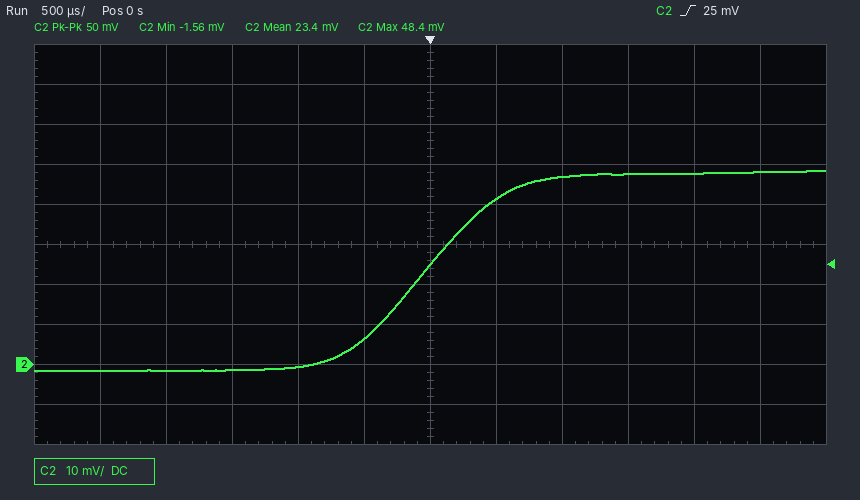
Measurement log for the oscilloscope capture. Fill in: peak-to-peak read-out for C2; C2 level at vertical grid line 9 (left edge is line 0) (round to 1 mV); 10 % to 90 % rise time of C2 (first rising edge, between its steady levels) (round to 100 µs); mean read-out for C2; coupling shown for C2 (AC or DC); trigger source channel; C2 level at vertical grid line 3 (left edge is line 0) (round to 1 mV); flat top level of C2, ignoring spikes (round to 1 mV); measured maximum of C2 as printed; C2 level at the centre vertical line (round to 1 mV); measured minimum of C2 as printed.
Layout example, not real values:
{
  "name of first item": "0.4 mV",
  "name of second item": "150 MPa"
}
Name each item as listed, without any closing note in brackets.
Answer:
{
  "peak-to-peak read-out for C2": "50 mV",
  "C2 level at vertical grid line 9 (left edge is line 0)": "48 mV",
  "10 % to 90 % rise time of C2 (first rising edge, between its steady levels)": "1.2 ms",
  "mean read-out for C2": "23.4 mV",
  "coupling shown for C2": "DC",
  "trigger source channel": "C2",
  "C2 level at vertical grid line 3 (left edge is line 0)": "-1 mV",
  "flat top level of C2, ignoring spikes": "48 mV",
  "measured maximum of C2 as printed": "48.4 mV",
  "C2 level at the centre vertical line": "25 mV",
  "measured minimum of C2 as printed": "-1.56 mV"
}
